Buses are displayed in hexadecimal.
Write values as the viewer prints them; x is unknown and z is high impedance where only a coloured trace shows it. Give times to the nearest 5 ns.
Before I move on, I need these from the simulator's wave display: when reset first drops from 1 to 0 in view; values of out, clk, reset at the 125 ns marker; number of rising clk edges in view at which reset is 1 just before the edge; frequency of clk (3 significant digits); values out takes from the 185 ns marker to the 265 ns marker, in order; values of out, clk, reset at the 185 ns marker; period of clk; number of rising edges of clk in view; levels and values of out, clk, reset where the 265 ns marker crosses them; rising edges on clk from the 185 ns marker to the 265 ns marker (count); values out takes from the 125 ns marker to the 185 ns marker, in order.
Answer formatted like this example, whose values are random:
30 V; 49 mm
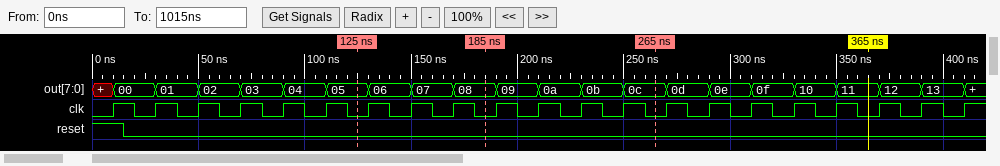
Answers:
15 ns; out=05, clk=0, reset=0; 1; 50.0 MHz; 08, 09, 0a, 0b, 0c; out=08, clk=0, reset=0; 20 ns; 21; out=0c, clk=0, reset=0; 4; 05, 06, 07, 08
